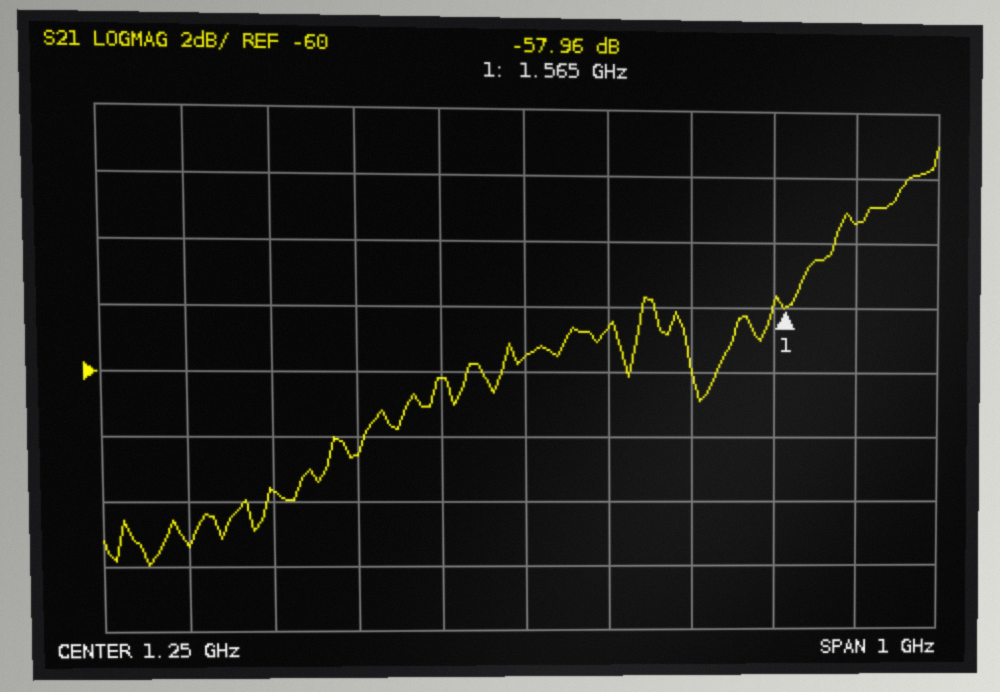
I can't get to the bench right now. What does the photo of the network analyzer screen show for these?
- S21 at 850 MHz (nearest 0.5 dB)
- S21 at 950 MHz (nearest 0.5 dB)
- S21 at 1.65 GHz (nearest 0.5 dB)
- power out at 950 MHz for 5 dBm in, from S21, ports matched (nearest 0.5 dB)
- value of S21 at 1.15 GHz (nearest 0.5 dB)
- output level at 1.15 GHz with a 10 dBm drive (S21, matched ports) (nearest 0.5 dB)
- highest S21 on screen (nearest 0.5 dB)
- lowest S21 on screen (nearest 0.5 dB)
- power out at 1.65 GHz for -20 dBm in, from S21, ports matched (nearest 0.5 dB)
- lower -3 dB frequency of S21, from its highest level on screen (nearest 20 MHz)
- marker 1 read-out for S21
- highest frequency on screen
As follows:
-65.5 dB
-63.5 dB
-55.5 dB
-58.5 dBm
-60.0 dB
-50.0 dBm
-53.0 dB
-66.0 dB
-75.5 dBm
1.62 GHz
-57.96 dB
1.75 GHz
